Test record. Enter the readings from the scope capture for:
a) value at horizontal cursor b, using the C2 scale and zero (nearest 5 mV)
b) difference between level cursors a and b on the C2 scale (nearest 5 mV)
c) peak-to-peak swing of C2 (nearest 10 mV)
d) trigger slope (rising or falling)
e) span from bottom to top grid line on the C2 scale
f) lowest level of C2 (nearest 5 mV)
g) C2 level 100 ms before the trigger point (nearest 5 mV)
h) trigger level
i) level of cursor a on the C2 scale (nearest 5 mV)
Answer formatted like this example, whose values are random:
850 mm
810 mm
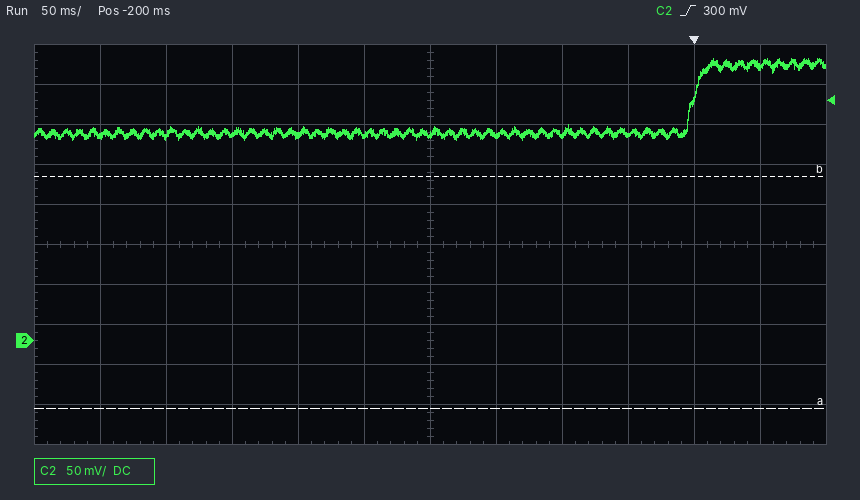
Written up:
205 mV
290 mV
100 mV
rising
500 mV
250 mV
260 mV
300 mV
-85 mV
